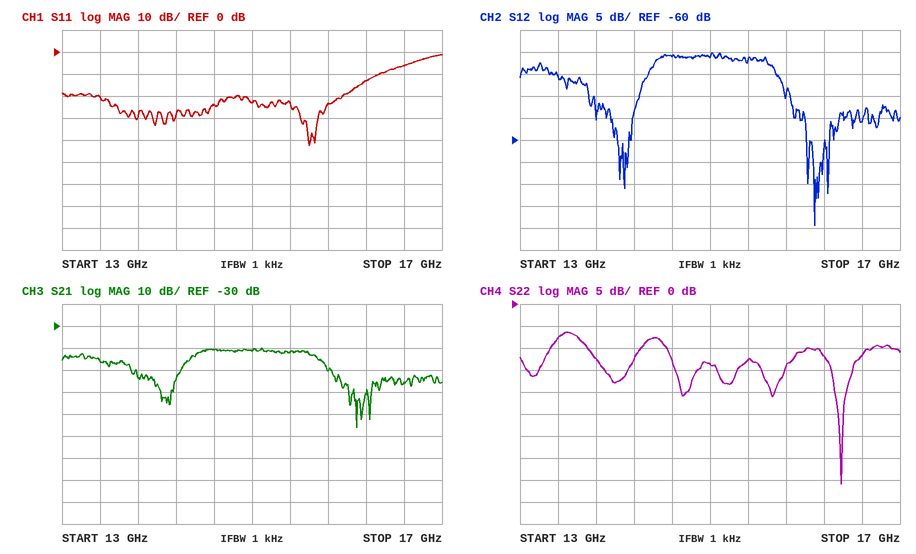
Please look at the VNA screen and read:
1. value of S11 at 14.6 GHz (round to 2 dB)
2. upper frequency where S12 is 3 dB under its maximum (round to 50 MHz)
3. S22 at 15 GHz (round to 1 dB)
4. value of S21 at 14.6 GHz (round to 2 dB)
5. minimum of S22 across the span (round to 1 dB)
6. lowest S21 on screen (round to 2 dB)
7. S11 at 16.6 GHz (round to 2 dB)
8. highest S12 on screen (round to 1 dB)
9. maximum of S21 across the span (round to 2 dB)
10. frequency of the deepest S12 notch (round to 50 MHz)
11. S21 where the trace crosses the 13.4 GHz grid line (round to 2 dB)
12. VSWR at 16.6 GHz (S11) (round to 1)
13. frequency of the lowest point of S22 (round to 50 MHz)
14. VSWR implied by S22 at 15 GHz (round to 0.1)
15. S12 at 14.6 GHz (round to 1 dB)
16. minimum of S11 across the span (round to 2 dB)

-24 dB
15.65 GHz
-14 dB
-40 dB
-41 dB
-76 dB
-6 dB
-40 dB
-40 dB
16.10 GHz
-46 dB
3
16.40 GHz
1.5
-41 dB
-42 dB
